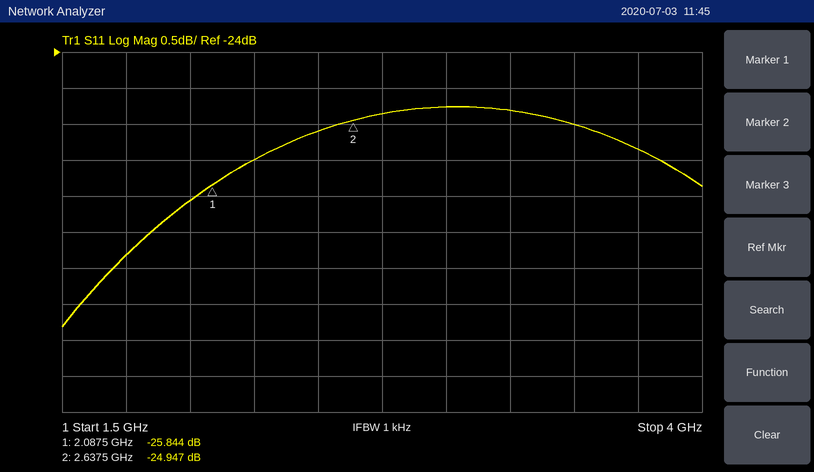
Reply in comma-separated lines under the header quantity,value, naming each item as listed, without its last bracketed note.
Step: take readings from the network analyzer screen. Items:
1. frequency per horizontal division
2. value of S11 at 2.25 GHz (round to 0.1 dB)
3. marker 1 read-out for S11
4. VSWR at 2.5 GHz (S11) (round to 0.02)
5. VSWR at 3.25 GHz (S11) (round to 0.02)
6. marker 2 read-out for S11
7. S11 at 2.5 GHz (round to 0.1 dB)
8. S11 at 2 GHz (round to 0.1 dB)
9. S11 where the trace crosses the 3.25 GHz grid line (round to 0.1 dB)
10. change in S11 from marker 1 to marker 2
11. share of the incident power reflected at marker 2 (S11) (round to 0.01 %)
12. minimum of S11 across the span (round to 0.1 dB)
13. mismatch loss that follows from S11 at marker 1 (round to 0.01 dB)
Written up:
quantity,value
frequency per horizontal division,250 MHz
value of S11 at 2.25 GHz,-25.5 dB
marker 1 read-out for S11,-25.844 dB
VSWR at 2.5 GHz (S11),1.12
VSWR at 3.25 GHz (S11),1.12
marker 2 read-out for S11,-24.947 dB
S11 at 2.5 GHz,-25.1 dB
S11 at 2 GHz,-26.1 dB
S11 where the trace crosses the 3.25 GHz grid line,-24.8 dB
change in S11 from marker 1 to marker 2,0.897 dB
share of the incident power reflected at marker 2 (S11),0.32 %
minimum of S11 across the span,-27.8 dB
mismatch loss that follows from S11 at marker 1,0.01 dB
